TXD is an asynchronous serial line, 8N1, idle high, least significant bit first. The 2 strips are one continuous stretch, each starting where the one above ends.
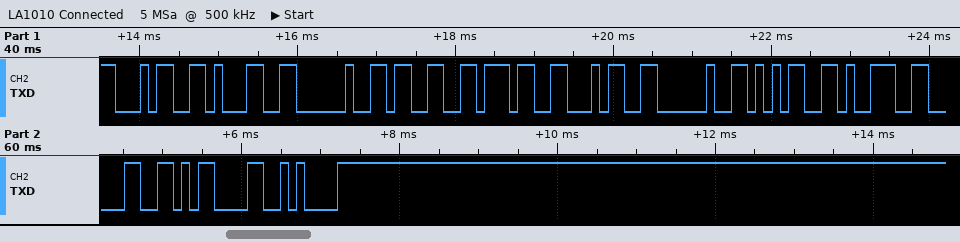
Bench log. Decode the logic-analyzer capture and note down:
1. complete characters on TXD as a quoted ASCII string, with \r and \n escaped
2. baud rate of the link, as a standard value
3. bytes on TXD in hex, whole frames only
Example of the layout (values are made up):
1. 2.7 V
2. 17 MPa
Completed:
1. "41 374 590\r\n"
2. 9600 baud
3. 34 31 20 33 37 34 20 35 39 30 0D 0A
